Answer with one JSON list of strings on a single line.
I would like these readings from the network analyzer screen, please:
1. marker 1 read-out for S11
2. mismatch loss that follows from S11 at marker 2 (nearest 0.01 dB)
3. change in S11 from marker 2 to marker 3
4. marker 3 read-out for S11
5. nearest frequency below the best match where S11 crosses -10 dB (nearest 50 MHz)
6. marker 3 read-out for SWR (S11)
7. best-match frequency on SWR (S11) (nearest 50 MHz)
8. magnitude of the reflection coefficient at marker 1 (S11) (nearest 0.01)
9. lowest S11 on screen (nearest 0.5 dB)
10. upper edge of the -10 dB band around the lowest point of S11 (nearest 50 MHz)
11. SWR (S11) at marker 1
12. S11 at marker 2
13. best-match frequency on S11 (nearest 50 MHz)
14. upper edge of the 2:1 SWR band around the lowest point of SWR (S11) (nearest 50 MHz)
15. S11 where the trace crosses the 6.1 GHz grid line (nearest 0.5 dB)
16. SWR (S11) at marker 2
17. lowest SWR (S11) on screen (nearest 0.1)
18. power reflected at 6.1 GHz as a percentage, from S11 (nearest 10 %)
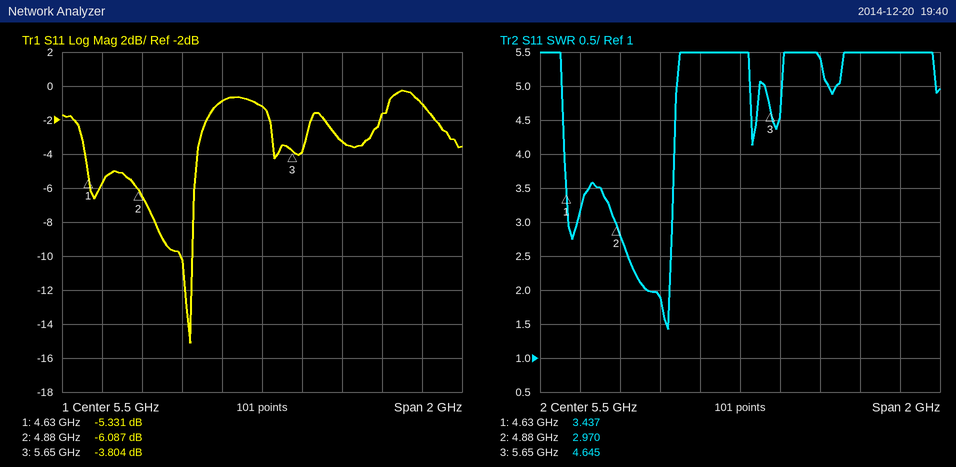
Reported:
["-5.331 dB", "1.23 dB", "2.283 dB", "-3.804 dB", "5.10 GHz", "4.645", "5.15 GHz", "0.54", "-15.0 dB", "5.15 GHz", "3.437", "-6.087 dB", "5.15 GHz", "5.15 GHz", "-1.5 dB", "2.970", "1.4", "70 %"]
